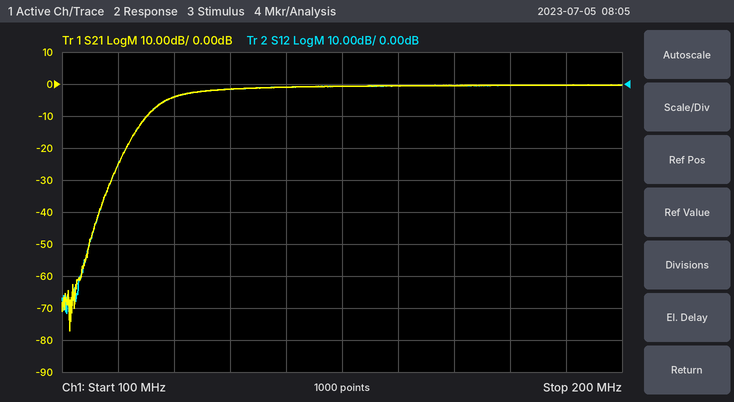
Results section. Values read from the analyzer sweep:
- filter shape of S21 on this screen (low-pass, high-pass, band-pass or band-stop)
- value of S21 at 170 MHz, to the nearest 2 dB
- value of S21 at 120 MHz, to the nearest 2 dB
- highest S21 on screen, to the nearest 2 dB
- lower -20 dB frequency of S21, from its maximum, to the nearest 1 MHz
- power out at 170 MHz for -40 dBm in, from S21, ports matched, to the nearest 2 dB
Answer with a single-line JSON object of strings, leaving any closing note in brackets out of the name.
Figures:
{"filter shape of S21 on this screen": "high-pass", "value of S21 at 170 MHz, to the nearest 2 dB": "0 dB", "value of S21 at 120 MHz, to the nearest 2 dB": "-4 dB", "highest S21 on screen, to the nearest 2 dB": "0 dB", "lower -20 dB frequency of S21, from its maximum, to the nearest 1 MHz": "111 MHz", "power out at 170 MHz for -40 dBm in, from S21, ports matched, to the nearest 2 dB": "-40 dBm"}
